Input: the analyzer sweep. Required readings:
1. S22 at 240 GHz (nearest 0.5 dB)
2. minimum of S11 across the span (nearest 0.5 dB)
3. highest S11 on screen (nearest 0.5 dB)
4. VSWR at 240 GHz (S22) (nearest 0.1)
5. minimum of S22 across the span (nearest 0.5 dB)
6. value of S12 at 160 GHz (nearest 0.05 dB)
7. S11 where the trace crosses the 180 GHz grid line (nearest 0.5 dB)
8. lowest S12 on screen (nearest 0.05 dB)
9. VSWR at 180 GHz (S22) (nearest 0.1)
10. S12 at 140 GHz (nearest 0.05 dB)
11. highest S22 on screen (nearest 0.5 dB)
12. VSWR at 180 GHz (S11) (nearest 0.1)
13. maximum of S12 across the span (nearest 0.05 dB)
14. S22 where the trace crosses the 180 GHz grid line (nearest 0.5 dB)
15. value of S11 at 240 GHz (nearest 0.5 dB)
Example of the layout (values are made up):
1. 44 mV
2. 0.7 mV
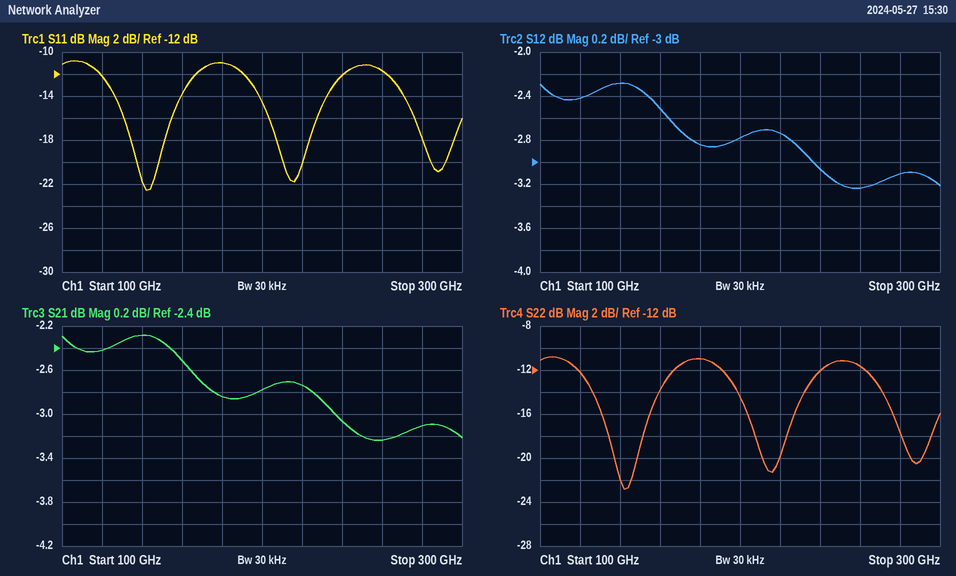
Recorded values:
1. -12.0 dB
2. -22.5 dB
3. -11.0 dB
4. 1.7
5. -23.0 dB
6. -2.50 dB
7. -11.0 dB
8. -3.25 dB
9. 1.8
10. -2.30 dB
11. -11.0 dB
12. 1.8
13. -2.30 dB
14. -11.0 dB
15. -12.0 dB
